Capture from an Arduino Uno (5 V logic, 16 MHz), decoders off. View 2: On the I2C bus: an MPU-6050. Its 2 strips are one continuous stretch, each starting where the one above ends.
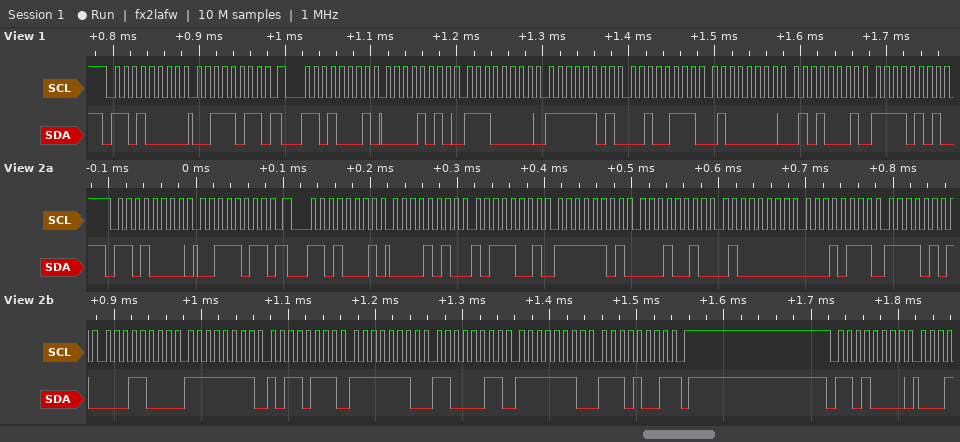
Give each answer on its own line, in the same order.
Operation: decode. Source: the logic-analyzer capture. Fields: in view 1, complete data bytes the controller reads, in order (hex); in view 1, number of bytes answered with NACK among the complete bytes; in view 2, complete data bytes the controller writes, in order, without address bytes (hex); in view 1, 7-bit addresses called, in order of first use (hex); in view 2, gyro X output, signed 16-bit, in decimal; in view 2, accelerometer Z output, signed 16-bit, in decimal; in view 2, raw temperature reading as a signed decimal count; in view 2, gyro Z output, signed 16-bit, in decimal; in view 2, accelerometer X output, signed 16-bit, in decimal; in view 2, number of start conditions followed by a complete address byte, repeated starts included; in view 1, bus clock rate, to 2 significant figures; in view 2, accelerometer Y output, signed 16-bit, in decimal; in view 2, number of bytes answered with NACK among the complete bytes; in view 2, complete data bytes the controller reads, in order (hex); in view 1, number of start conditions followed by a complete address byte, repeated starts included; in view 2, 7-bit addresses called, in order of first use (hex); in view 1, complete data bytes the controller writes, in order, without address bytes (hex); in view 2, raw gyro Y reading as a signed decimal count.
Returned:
0A E0 FD 27 40 51 F5
0
3B
0x68
-73
16407
-2792
-279
2745
3
100 kHz
-750
1
0A B9 FD 12 40 17 F5 18 FF B7 FE C3 FE E9
2
0x68
3B
-317
